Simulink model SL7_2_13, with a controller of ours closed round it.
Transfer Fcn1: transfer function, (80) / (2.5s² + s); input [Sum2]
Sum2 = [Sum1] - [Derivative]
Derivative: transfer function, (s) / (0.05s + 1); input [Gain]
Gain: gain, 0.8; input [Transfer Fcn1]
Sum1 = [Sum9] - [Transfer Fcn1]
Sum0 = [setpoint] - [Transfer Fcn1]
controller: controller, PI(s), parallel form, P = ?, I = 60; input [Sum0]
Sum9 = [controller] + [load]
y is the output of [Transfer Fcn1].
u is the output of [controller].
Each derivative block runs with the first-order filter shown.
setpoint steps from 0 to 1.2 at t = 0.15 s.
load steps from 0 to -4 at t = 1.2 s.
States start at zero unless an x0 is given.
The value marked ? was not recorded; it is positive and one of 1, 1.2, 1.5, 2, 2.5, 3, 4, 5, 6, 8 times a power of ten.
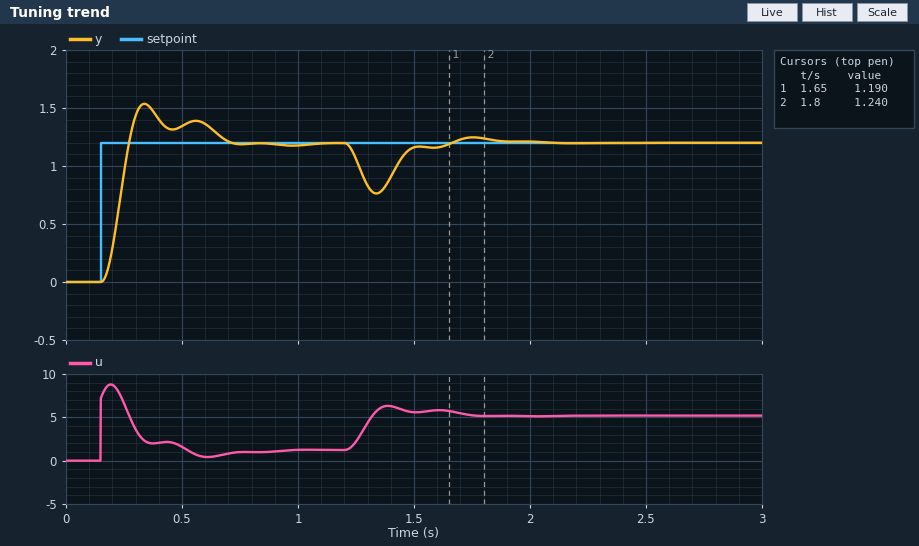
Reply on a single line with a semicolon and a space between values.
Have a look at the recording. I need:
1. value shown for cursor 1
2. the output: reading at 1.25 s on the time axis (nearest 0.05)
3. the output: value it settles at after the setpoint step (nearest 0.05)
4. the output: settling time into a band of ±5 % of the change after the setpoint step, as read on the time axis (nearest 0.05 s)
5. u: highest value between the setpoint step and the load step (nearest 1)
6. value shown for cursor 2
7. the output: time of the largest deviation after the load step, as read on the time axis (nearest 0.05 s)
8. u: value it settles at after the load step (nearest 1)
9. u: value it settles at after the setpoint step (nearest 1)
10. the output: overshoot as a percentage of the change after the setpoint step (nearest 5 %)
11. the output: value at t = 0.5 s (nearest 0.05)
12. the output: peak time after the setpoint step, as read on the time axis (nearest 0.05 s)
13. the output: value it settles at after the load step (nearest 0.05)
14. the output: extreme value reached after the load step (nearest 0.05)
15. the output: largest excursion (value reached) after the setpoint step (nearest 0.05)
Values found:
1.190; 1.05; 1.20; 0.65 s; 9; 1.240; 1.35 s; 5; 1; 30 %; 1.35; 0.35 s; 1.20; 0.75; 1.55
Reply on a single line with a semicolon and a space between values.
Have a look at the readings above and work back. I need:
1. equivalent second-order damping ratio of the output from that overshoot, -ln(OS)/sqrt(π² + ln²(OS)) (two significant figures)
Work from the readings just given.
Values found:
0.36
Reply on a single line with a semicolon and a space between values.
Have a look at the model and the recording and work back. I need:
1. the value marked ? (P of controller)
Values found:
6
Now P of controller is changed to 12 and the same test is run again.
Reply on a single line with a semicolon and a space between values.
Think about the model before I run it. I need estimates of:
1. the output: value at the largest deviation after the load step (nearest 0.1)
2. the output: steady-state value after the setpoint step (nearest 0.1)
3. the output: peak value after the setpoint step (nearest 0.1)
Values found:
0.9; 1.2; 1.6
